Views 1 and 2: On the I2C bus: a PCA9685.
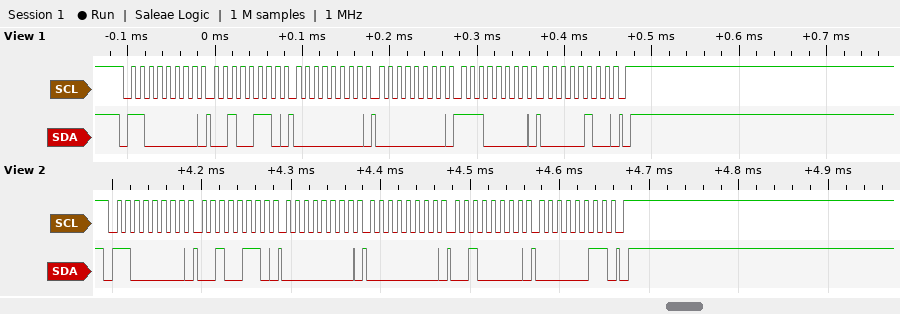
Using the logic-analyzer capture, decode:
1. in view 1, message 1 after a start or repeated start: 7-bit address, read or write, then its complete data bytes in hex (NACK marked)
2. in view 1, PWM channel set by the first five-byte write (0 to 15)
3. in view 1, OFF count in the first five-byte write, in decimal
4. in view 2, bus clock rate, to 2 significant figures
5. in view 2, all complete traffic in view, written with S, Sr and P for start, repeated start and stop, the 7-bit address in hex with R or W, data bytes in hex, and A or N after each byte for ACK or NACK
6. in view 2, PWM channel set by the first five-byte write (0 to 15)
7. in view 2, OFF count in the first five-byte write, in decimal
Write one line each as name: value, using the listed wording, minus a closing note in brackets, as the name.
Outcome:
in view 1, message 1 after a start or repeated start: 7-bit address, read or write, then its complete data bytes in hex: 0x60 write: 26 00 00 E0 04
in view 1, PWM channel set by the first five-byte write: 8
in view 1, OFF count in the first five-byte write, in decimal: 1248
in view 2, bus clock rate, to 2 significant figures: 100 kHz
in view 2, all complete traffic in view, written with S, Sr and P for start, repeated start and stop, the 7-bit address in hex with R or W, data bytes in hex, and A or N after each byte for ACK or NACK: S 60W A 26 A 00 A 00 A 20 A 03 A P
in view 2, PWM channel set by the first five-byte write: 8
in view 2, OFF count in the first five-byte write, in decimal: 800
